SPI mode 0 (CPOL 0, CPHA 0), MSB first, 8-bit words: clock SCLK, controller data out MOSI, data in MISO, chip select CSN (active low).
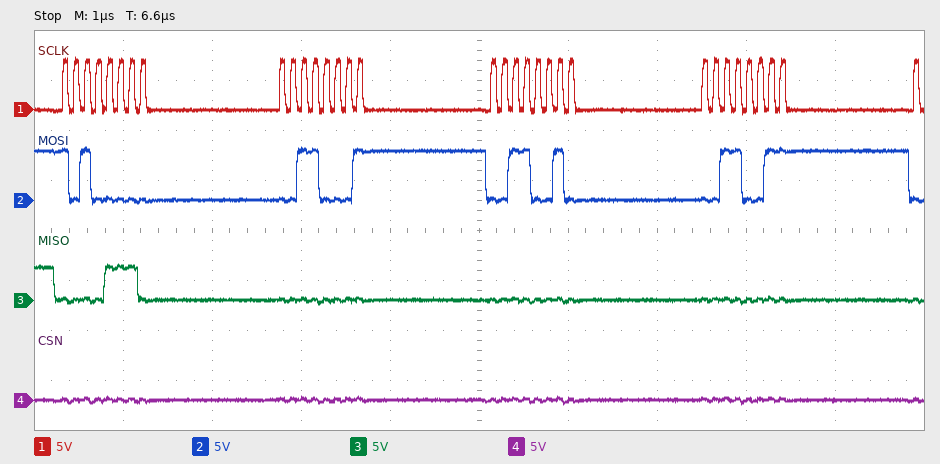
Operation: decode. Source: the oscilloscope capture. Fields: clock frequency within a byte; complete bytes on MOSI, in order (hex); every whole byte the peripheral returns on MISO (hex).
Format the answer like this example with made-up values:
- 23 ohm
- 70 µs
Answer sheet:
- 8 MHz
- 0xA0 0x31 0x32 0x33
- 0x0E 0x00 0x00 0x00
